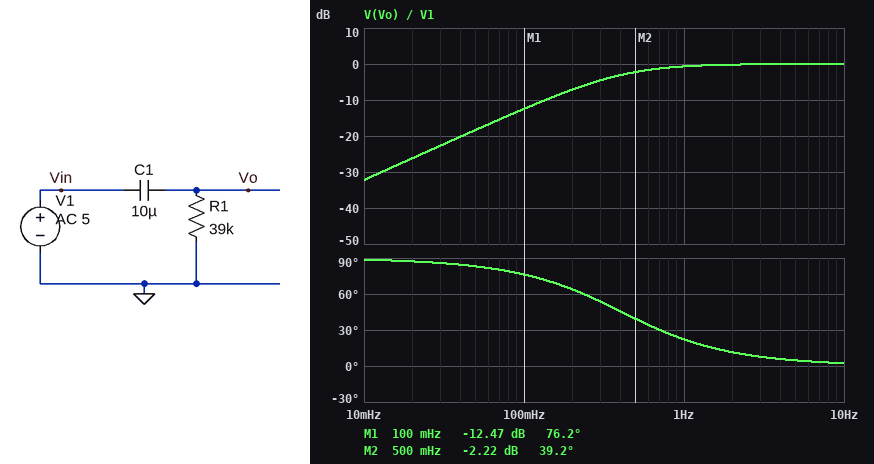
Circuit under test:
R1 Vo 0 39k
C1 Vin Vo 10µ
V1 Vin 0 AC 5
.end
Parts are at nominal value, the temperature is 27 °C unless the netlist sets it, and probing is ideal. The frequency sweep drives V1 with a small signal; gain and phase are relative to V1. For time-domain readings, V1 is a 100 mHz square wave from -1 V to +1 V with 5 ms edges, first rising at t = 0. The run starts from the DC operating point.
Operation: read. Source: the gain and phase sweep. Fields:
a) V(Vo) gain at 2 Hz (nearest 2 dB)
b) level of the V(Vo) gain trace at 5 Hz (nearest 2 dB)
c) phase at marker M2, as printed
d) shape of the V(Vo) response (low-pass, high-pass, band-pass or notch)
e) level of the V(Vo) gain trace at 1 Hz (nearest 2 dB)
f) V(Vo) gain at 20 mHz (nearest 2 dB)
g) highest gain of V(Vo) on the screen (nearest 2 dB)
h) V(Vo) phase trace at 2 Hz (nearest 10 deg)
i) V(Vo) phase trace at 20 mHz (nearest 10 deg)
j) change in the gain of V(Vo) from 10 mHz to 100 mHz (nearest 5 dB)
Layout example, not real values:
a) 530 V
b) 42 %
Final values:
a) 0 dB
b) 0 dB
c) 39.2 deg
d) high-pass
e) 0 dB
f) -26 dB
g) 0 dB
h) 10 deg
i) 90 deg
j) 20 dB
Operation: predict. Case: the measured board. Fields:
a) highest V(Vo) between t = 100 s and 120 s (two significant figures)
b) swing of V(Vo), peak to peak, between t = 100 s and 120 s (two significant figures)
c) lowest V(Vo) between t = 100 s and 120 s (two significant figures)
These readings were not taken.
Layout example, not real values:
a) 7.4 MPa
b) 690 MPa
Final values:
a) 2.0 V
b) 4.0 V
c) -2.0 V
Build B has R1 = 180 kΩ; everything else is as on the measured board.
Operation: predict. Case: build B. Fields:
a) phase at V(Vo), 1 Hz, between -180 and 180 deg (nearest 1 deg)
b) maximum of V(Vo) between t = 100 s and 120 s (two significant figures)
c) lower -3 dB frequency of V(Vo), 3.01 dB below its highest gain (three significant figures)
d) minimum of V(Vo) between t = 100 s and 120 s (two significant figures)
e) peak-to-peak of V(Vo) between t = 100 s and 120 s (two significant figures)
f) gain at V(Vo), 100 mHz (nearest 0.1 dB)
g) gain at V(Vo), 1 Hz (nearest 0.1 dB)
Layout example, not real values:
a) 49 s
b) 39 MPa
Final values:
a) 5 deg
b) 1.9 V
c) 88.4 mHz
d) -1.9 V
e) 3.8 V
f) -2.5 dB
g) 0 dB
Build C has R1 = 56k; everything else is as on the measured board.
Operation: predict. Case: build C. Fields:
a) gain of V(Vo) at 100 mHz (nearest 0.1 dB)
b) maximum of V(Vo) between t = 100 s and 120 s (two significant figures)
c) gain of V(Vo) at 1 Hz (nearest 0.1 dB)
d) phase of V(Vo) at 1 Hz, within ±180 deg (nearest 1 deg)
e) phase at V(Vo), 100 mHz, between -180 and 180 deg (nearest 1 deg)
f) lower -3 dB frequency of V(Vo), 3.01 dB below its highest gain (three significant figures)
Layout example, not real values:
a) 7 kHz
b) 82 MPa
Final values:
a) -9.6 dB
b) 2.0 V
c) -0.3 dB
d) 16 deg
e) 71 deg
f) 284 mHz
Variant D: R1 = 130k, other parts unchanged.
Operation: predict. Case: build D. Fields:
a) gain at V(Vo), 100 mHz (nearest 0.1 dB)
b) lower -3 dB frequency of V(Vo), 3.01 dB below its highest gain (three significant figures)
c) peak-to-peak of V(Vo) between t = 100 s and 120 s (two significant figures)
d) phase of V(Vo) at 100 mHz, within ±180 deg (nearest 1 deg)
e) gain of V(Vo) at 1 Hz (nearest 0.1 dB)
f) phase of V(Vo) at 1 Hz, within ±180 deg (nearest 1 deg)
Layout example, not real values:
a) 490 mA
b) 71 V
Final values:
a) -4.0 dB
b) 122 mHz
c) 3.9 V
d) 51 deg
e) -0.1 dB
f) 7 deg
